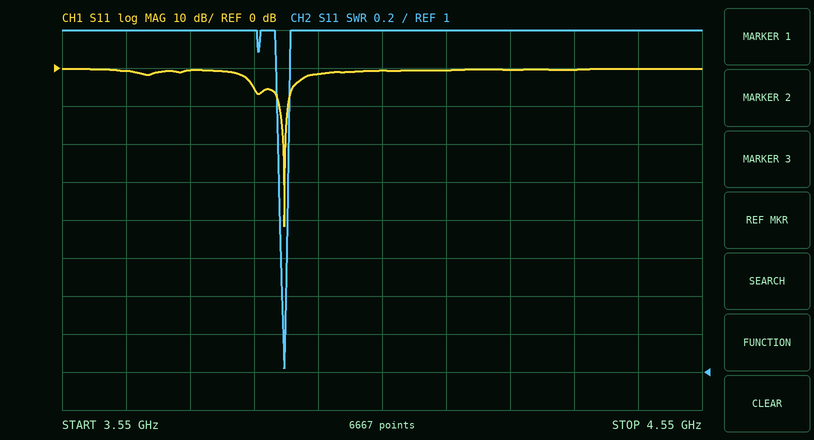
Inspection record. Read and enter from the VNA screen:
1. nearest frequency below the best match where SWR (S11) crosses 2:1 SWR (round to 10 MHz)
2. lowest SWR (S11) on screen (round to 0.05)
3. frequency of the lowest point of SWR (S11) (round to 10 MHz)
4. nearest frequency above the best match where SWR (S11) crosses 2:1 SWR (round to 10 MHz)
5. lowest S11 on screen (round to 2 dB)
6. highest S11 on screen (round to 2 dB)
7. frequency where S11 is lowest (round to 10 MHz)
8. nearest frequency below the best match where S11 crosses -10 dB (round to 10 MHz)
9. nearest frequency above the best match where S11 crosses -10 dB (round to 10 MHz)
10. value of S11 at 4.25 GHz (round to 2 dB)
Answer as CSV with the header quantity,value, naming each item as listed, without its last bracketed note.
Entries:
quantity,value
nearest frequency below the best match where SWR (S11) crosses 2:1 SWR,3.89 GHz
lowest SWR (S11) on screen,1.00
frequency of the lowest point of SWR (S11),3.90 GHz
nearest frequency above the best match where SWR (S11) crosses 2:1 SWR,3.90 GHz
lowest S11 on screen,-42 dB
highest S11 on screen,0 dB
frequency where S11 is lowest,3.90 GHz
nearest frequency below the best match where S11 crosses -10 dB,3.89 GHz
nearest frequency above the best match where S11 crosses -10 dB,3.90 GHz
value of S11 at 4.25 GHz,0 dB
